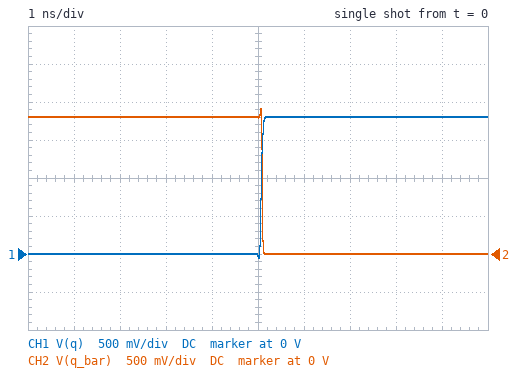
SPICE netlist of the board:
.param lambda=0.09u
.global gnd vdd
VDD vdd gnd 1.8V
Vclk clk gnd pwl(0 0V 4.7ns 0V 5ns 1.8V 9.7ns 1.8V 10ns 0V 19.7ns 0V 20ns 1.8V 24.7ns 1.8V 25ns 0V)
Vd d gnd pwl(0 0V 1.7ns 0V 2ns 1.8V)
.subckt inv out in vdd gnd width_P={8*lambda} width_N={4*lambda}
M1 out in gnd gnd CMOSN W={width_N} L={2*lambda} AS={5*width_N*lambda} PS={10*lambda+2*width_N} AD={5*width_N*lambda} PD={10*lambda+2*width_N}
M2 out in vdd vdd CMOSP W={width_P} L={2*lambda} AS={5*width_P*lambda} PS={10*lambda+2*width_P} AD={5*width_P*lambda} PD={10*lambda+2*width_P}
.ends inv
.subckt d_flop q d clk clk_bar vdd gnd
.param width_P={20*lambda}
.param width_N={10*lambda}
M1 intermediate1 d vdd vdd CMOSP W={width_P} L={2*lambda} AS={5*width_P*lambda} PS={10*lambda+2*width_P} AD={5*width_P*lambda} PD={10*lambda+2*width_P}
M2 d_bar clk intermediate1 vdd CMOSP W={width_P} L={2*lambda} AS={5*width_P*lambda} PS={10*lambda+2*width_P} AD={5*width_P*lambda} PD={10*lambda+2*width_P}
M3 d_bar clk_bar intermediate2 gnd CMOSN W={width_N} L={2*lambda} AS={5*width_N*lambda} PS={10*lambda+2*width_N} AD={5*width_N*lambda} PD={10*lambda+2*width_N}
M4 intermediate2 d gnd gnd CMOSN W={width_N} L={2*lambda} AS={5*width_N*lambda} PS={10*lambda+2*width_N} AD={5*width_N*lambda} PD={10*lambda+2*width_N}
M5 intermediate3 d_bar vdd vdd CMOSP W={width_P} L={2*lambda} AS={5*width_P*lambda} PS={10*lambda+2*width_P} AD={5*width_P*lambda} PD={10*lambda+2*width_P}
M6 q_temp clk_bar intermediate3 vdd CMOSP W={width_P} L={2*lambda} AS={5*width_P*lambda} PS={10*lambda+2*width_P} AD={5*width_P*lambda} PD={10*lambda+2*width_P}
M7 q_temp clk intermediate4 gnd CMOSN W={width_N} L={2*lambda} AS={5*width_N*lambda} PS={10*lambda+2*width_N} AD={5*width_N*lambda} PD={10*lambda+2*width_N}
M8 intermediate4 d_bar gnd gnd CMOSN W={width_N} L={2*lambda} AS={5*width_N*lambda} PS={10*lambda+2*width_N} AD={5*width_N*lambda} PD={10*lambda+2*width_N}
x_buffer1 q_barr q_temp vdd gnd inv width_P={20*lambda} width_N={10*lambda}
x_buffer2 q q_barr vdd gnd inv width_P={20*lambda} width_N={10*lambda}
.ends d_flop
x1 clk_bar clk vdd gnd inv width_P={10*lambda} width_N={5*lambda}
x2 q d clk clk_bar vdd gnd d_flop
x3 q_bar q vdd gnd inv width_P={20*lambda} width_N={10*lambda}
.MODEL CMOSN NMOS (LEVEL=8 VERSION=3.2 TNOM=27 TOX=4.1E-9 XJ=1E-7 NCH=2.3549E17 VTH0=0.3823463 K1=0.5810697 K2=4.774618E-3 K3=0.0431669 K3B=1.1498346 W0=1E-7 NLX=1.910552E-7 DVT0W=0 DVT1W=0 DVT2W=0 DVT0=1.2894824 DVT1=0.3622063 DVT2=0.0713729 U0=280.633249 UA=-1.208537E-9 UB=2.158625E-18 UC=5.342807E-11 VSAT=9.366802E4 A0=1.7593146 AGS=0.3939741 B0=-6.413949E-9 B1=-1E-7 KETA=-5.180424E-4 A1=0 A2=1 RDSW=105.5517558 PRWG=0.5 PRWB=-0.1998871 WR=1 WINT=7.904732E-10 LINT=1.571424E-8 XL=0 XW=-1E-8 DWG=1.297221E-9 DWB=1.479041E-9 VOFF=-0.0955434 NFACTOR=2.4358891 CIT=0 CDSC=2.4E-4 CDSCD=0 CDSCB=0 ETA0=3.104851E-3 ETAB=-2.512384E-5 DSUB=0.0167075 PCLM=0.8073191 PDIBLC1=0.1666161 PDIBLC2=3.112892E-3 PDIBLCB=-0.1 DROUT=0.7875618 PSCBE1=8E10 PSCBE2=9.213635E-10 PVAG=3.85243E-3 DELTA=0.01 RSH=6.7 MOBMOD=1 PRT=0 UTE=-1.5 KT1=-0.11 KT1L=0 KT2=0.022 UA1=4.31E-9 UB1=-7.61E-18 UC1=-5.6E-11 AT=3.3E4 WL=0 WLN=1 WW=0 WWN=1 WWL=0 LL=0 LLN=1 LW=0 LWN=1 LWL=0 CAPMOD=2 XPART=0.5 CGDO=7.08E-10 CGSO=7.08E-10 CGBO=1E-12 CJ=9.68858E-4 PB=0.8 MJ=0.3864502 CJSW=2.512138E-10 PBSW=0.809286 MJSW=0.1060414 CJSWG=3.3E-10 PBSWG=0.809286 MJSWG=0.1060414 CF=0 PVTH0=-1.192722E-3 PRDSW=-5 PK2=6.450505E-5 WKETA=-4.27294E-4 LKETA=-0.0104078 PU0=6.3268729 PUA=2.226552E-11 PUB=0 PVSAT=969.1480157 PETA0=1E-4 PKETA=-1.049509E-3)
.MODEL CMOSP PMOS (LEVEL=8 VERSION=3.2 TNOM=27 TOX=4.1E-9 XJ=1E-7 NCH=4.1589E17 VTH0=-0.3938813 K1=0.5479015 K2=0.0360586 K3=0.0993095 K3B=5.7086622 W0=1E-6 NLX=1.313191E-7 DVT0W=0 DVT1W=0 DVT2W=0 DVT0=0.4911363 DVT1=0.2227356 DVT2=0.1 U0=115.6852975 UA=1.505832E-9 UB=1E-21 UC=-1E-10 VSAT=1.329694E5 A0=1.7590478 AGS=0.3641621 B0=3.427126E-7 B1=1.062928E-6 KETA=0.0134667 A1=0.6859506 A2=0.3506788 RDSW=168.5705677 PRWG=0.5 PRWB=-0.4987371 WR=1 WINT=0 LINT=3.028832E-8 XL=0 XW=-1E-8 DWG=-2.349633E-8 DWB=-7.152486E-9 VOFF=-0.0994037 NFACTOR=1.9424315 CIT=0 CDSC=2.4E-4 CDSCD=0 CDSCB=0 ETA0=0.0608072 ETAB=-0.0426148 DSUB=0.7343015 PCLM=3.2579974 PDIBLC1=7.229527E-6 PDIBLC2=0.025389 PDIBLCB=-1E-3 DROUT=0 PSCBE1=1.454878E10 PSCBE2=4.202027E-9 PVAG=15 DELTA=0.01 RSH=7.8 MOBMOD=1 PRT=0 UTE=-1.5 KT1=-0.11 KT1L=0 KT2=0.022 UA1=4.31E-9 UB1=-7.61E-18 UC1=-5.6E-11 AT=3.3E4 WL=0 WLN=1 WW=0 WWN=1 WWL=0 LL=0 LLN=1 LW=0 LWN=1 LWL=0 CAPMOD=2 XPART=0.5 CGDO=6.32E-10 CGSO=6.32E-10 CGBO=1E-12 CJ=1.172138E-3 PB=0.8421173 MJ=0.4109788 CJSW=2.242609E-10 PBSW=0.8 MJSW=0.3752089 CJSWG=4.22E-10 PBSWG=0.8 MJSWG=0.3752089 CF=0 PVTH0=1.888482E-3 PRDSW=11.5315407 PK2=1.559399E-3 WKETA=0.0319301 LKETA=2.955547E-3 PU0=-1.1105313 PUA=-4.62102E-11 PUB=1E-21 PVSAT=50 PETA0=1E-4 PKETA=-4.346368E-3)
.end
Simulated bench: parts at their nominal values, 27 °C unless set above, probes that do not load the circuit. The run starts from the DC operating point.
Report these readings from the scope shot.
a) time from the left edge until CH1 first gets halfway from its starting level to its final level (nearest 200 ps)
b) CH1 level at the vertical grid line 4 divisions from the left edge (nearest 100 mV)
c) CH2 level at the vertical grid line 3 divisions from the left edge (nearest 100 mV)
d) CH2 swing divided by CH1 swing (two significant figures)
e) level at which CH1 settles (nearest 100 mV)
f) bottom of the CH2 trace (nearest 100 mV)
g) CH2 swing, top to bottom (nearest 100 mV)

5.0 ns
0 V
1.8 V
1.0
1.8 V
0 V
1.9 V
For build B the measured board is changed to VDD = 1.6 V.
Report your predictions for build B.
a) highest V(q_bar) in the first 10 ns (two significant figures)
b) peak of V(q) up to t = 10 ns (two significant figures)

1.7 V
1.6 V
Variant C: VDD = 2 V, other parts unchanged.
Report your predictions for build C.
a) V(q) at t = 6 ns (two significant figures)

2.0 V
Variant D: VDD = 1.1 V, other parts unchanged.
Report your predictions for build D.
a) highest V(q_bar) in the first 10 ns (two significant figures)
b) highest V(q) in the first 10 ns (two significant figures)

1.2 V
1.1 V
